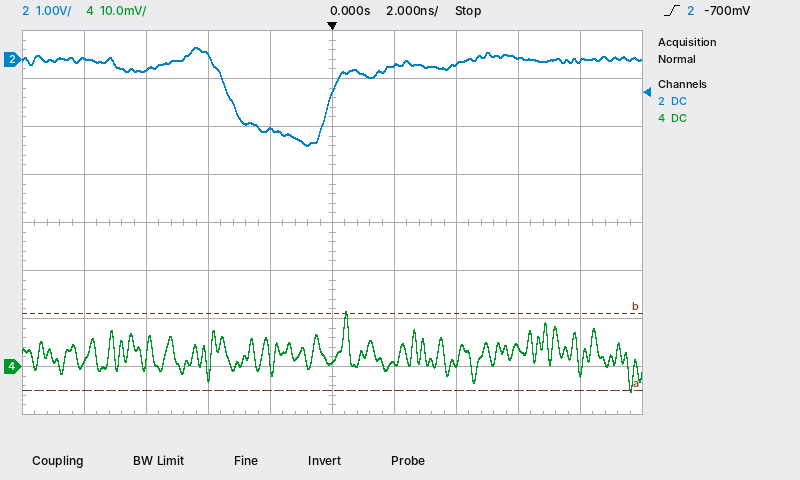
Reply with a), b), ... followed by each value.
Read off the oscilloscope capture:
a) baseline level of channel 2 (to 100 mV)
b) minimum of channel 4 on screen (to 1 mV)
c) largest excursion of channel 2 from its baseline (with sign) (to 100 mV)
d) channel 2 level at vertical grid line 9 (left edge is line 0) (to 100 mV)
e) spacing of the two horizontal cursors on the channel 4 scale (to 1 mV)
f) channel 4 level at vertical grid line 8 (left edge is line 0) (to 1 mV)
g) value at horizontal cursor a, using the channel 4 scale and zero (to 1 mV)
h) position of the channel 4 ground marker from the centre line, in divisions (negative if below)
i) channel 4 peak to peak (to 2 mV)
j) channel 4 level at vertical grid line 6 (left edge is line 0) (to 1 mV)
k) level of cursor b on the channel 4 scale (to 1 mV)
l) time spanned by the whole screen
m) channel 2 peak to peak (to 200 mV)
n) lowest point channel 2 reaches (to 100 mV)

a) 0.0 V
b) -5 mV
c) -1.8 V
d) 0.0 V
e) 16 mV
f) 4 mV
g) -5 mV
h) -3.0 div
i) 16 mV
j) 1 mV
k) 11 mV
l) 20 ns
m) 2.0 V
n) -1.8 V
